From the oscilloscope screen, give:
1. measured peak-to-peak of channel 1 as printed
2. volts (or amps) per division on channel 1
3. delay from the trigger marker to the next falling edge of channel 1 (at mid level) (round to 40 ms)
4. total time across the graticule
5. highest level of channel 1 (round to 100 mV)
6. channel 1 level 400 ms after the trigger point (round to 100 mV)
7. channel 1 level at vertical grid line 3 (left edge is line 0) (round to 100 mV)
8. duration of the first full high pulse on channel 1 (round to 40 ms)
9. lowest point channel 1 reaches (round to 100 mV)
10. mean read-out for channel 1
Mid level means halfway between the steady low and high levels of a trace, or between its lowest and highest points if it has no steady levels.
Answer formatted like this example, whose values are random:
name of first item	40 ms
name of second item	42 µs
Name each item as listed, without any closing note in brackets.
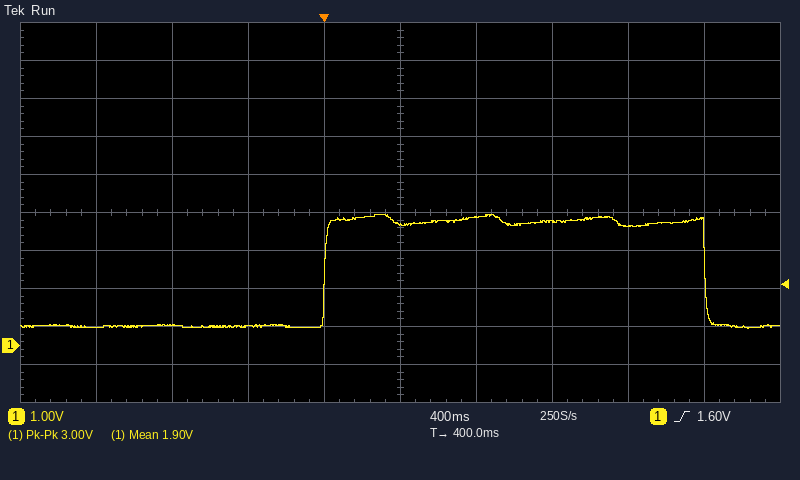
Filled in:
measured peak-to-peak of channel 1 as printed	3.00 V
volts (or amps) per division on channel 1	1 V
delay from the trigger marker to the next falling edge of channel 1 (at mid level)	2.00 s
total time across the graticule	4 s
highest level of channel 1	3.4 V
channel 1 level 400 ms after the trigger point	3.2 V
channel 1 level at vertical grid line 3 (left edge is line 0)	500 mV
duration of the first full high pulse on channel 1	2.00 s
lowest point channel 1 reaches	400 mV
mean read-out for channel 1	1.90 V
